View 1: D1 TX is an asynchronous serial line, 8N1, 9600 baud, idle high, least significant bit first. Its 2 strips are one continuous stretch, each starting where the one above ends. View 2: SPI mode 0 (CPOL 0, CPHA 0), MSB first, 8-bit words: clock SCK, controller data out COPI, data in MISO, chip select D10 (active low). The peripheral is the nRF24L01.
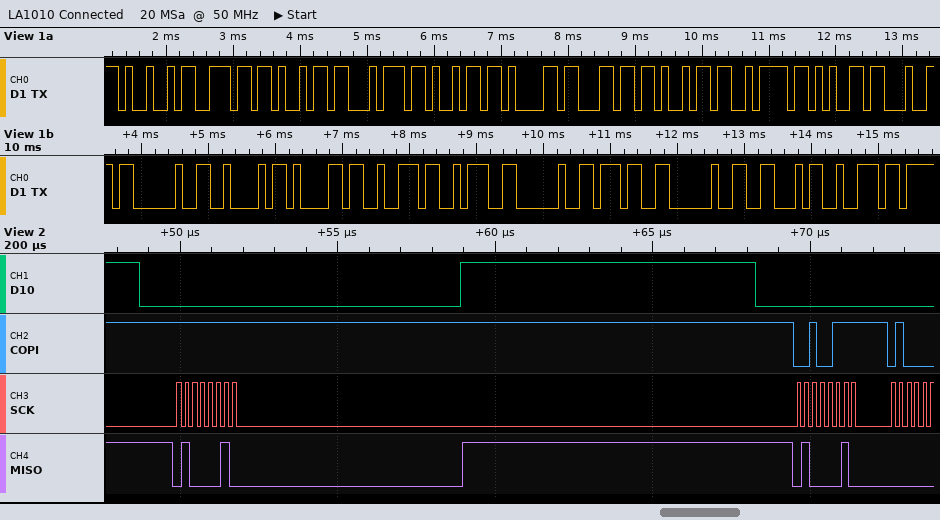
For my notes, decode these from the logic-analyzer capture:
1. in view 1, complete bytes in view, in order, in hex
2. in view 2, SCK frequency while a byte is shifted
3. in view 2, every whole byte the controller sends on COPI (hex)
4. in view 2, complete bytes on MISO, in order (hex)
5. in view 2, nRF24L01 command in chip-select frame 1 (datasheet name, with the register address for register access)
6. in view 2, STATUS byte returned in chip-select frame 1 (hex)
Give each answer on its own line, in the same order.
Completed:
0x49 0x6E 0x69 0x74 0x69 0x61 0x6C 0x69 0x7A 0x65 0x64 0x20 0x42 0x61 0x72 0x3A 0x20 0x37 0x20 0x46 0x72
4 MHz
FF 27
42 42
NOP
0x42
